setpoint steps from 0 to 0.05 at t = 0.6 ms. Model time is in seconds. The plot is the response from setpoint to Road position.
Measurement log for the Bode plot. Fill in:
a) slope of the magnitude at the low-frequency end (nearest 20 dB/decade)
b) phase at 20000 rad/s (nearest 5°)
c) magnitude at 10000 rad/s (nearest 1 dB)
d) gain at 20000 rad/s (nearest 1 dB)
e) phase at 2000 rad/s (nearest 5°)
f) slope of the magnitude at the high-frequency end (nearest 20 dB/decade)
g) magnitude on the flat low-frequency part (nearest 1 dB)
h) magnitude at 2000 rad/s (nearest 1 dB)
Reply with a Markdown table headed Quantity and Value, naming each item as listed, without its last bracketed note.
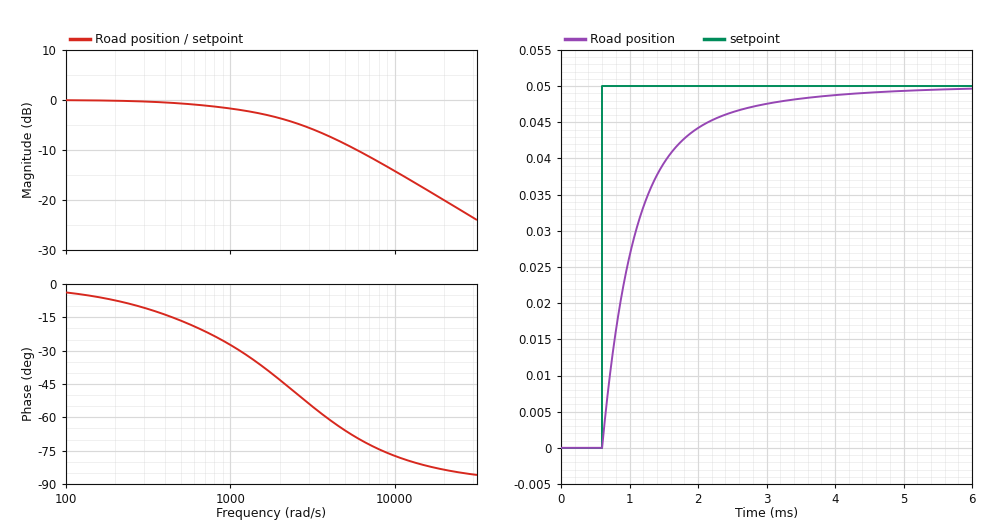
| Quantity | Value |
|---|---|
| slope of the magnitude at the low-frequency end | 0 dB/decade |
| phase at 20000 rad/s | -85° |
| magnitude at 10000 rad/s | -14 dB |
| gain at 20000 rad/s | -20 dB |
| phase at 2000 rad/s | -45° |
| slope of the magnitude at the high-frequency end | -20 dB/decade |
| magnitude on the flat low-frequency part | 0 dB |
| magnitude at 2000 rad/s | -4 dB |
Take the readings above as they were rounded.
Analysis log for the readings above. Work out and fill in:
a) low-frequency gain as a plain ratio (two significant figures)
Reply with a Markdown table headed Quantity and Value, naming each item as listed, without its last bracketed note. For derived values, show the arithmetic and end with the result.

| Quantity | Value |
|---|---|
| low-frequency gain as a plain ratio | 10^(0 / 20) = 1.0 |
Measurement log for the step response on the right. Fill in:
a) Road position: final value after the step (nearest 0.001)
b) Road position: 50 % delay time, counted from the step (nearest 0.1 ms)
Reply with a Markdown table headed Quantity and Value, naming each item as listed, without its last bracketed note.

| Quantity | Value |
|---|---|
| Road position: final value after the step | 0.050 |
| Road position: 50 % delay time, counted from the step | 0.4 ms |
